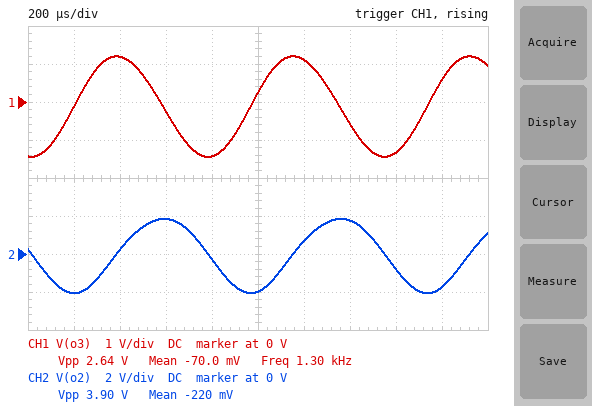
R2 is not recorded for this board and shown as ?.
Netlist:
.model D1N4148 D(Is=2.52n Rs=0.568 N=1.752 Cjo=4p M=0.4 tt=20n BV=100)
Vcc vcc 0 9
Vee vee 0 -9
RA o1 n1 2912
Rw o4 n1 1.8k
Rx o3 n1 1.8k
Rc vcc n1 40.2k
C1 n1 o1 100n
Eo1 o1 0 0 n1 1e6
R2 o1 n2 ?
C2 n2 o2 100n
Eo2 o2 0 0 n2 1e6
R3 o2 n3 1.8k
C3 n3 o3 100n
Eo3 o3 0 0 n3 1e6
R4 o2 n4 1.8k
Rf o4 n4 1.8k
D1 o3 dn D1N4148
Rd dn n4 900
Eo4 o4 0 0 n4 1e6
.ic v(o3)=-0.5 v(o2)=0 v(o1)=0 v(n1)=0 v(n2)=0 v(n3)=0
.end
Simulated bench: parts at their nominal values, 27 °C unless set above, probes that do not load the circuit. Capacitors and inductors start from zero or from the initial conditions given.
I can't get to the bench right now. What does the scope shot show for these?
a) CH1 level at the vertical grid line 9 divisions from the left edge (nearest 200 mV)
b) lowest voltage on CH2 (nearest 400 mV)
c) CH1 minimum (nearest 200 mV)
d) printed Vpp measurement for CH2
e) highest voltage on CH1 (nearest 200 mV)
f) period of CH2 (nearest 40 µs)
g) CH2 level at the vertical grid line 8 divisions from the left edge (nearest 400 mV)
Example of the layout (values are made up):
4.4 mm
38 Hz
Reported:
600 mV
-2.0 V
-1.4 V
3.90 V
1.2 V
760 µs
-800 mV
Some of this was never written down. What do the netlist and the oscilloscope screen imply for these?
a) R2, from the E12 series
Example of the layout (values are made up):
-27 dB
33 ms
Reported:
820 Ω
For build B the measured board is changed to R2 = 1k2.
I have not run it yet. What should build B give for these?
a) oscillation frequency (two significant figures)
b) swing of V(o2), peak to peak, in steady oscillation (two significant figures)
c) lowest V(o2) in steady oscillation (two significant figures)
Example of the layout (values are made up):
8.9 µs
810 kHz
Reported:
1.1 kHz
3.3 V
-1.7 V
